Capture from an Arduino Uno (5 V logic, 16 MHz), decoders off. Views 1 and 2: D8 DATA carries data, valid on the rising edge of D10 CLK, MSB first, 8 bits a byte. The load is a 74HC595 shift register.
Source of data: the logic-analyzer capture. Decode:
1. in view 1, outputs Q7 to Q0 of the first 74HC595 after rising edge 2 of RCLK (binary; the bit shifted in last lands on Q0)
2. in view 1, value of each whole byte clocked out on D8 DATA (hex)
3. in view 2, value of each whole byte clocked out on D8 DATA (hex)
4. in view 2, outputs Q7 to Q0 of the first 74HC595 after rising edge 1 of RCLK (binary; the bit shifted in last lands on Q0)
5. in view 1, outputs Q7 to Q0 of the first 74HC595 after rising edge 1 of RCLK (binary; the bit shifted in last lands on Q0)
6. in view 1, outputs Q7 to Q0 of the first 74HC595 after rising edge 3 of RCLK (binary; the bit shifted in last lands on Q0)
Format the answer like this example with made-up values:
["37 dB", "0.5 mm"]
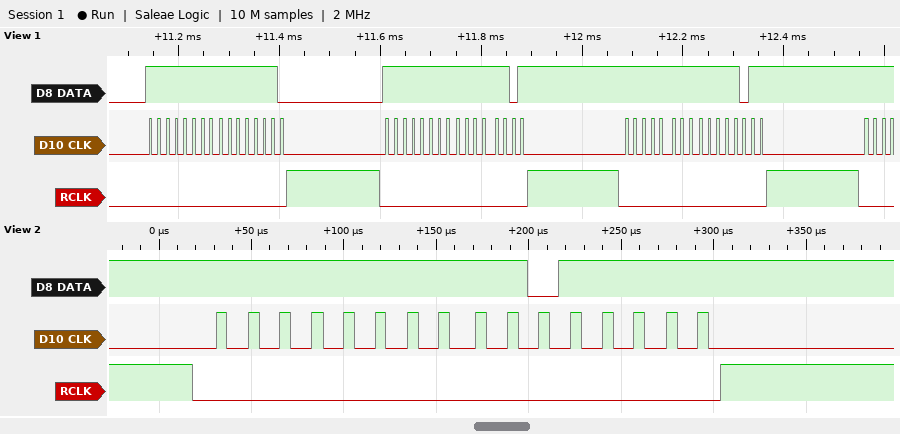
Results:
["11111101", "0xFF 0xFE 0xFF 0xFD 0xFF 0xFB", "FF DF", "11011111", "11111110", "11111011"]
